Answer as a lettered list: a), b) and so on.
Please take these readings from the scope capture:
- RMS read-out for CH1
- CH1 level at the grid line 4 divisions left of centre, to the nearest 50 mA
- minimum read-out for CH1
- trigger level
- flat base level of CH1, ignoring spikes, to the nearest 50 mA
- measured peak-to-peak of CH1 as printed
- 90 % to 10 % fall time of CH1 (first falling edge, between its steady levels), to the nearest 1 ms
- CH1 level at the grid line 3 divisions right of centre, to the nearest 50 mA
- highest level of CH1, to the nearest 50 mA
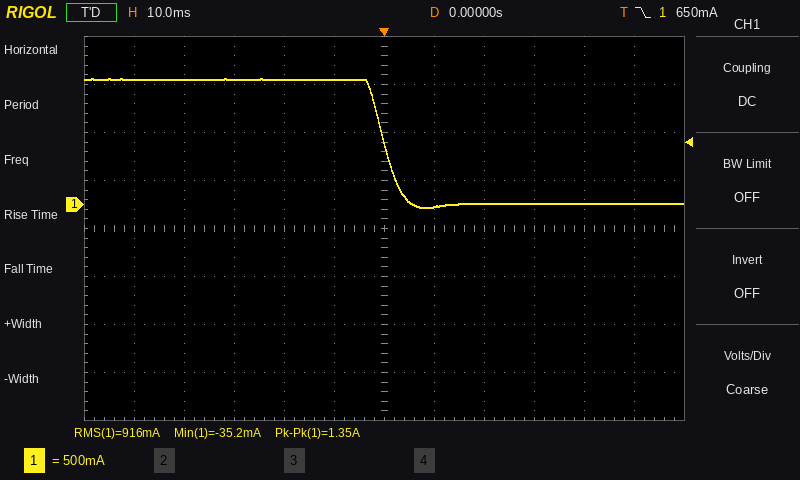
a) 916 mA
b) 1.30 A
c) -35.2 mA
d) 650 mA
e) 0 mA
f) 1.35 A
g) 6 ms
h) 0 mA
i) 1.30 A
